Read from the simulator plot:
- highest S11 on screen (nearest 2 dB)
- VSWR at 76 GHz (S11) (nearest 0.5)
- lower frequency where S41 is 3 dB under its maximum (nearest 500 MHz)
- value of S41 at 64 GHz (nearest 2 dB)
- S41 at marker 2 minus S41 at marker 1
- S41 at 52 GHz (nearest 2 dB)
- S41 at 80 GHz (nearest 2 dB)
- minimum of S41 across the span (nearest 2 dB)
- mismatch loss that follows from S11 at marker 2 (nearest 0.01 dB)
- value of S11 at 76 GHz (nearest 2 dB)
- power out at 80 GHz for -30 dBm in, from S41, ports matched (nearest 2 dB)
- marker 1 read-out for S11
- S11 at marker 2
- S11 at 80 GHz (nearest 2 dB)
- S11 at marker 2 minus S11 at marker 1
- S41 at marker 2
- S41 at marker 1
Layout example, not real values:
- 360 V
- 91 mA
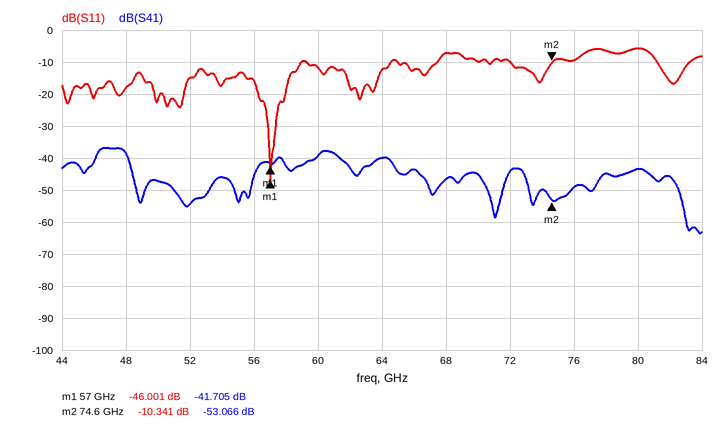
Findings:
- -6 dB
- 2.0
- 46.0 GHz
- -40 dB
- -11.361 dB
- -54 dB
- -44 dB
- -64 dB
- 0.42 dB
- -10 dB
- -74 dBm
- -46.001 dB
- -10.341 dB
- -6 dB
- 35.660 dB
- -53.066 dB
- -41.705 dB
